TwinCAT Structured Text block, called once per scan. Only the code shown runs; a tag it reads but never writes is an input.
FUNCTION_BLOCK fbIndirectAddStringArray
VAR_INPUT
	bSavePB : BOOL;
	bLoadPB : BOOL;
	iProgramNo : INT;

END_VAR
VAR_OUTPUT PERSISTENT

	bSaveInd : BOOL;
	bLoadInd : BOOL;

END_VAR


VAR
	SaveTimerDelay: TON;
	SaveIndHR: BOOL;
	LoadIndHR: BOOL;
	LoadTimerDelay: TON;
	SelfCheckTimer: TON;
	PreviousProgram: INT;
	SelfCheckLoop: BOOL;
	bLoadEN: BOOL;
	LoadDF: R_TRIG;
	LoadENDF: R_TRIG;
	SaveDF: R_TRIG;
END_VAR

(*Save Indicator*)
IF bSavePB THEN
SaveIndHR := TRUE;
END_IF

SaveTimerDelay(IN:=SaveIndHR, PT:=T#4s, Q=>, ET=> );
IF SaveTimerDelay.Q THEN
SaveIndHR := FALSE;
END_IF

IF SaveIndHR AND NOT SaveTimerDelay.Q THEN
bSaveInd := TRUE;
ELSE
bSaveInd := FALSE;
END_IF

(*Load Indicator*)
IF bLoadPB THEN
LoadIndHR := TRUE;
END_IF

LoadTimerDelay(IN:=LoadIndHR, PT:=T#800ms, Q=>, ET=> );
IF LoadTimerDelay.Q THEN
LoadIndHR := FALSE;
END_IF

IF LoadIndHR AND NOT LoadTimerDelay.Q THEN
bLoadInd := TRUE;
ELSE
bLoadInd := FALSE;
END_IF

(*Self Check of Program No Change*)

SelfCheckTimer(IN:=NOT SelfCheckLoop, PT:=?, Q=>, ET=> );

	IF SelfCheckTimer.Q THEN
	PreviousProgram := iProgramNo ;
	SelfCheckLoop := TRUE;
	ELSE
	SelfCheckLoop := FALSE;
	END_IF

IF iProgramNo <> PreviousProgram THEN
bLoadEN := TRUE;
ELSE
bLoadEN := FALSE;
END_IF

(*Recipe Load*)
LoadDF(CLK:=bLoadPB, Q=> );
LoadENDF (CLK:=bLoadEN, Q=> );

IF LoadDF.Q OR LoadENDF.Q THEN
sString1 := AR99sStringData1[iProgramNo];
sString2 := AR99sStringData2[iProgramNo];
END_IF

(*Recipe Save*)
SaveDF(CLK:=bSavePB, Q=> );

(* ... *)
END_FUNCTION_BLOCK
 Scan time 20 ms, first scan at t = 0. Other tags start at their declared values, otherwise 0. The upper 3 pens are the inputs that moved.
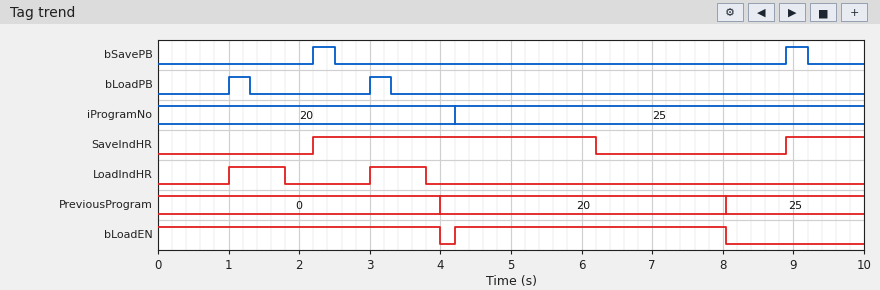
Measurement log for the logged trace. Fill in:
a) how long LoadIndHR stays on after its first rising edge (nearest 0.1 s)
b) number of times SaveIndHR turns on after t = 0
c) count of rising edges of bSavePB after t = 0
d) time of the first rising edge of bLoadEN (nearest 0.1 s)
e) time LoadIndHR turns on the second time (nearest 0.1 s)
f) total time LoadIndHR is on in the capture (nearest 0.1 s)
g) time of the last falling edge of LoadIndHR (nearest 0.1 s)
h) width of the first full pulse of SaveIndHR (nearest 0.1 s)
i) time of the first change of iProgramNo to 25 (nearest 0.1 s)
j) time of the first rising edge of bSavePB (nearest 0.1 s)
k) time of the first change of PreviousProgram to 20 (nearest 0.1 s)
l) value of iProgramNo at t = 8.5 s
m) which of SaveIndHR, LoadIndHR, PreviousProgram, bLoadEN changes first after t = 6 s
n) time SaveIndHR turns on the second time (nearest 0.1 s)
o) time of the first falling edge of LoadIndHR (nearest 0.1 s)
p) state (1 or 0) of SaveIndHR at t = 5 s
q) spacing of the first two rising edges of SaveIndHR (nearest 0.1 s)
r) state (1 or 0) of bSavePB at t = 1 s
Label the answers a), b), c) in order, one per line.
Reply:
a) 0.8 s
b) 2
c) 2
d) 4.2 s
e) 3.0 s
f) 1.6 s
g) 3.8 s
h) 4.0 s
i) 4.2 s
j) 2.2 s
k) 4.0 s
l) 25
m) SaveIndHR
n) 8.9 s
o) 1.8 s
p) 1
q) 6.7 s
r) 0
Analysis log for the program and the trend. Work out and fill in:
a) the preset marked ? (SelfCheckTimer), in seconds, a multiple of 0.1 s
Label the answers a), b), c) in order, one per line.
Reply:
a) 4.0 s
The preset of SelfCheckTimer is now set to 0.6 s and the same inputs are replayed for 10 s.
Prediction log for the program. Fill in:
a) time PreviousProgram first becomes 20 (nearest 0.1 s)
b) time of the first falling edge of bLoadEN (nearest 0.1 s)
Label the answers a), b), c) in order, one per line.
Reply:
a) 0.6 s
b) 0.6 s
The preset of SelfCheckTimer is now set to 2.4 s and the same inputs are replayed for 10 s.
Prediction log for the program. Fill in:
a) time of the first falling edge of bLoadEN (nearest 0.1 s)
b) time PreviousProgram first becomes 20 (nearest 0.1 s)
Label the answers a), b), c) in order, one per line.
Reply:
a) 2.4 s
b) 2.4 s
